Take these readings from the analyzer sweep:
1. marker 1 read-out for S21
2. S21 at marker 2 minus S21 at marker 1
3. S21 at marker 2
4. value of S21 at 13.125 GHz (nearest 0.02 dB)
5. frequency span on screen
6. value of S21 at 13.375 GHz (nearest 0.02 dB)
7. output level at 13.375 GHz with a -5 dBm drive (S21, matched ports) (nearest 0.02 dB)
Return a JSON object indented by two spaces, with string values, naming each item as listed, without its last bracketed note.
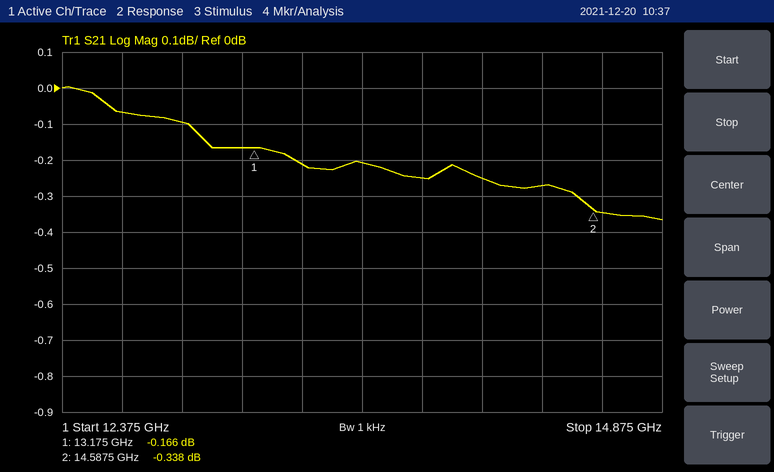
{
  "marker 1 read-out for S21": "-0.166 dB",
  "S21 at marker 2 minus S21 at marker 1": "-0.172 dB",
  "S21 at marker 2": "-0.338 dB",
  "value of S21 at 13.125 GHz": "-0.16 dB",
  "frequency span on screen": "2.5 GHz",
  "value of S21 at 13.375 GHz": "-0.22 dB",
  "output level at 13.375 GHz with a -5 dBm drive (S21, matched ports)": "-5.22 dBm"
}
